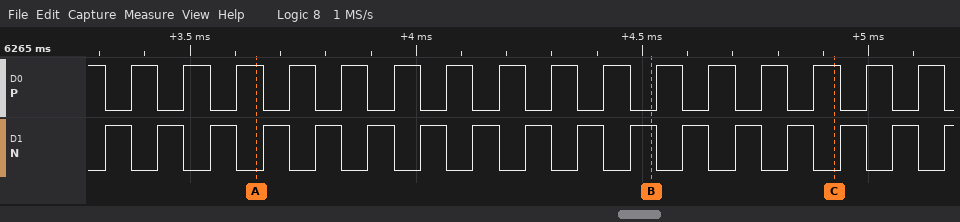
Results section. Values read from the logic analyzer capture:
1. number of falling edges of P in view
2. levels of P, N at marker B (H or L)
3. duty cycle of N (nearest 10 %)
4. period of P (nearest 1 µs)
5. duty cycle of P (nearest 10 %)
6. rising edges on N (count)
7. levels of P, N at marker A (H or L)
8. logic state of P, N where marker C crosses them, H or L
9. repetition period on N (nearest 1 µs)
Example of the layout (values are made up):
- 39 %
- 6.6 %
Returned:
- 17
- P=L, N=H
- 50 %
- 116 µs
- 50 %
- 17
- P=H, N=L
- P=H, N=L
- 116 µs
